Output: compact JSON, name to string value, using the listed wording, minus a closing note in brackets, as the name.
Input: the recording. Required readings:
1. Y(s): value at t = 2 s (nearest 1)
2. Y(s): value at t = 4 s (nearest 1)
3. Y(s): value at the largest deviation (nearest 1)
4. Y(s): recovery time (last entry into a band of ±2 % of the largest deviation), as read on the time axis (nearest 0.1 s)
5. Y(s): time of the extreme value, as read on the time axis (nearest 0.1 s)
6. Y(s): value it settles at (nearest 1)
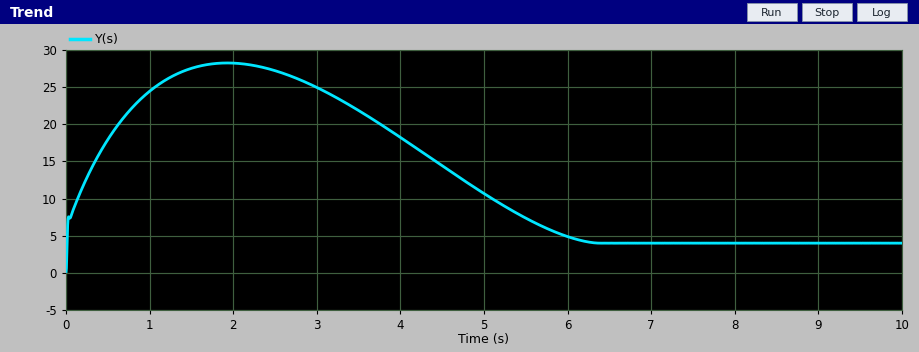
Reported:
{"Y(s): value at t = 2 s": "28", "Y(s): value at t = 4 s": "18", "Y(s): value at the largest deviation": "28", "Y(s): recovery time (last entry into a band of ±2 % of the largest deviation), as read on the time axis": "6.1 s", "Y(s): time of the extreme value, as read on the time axis": "1.9 s", "Y(s): value it settles at": "4"}
